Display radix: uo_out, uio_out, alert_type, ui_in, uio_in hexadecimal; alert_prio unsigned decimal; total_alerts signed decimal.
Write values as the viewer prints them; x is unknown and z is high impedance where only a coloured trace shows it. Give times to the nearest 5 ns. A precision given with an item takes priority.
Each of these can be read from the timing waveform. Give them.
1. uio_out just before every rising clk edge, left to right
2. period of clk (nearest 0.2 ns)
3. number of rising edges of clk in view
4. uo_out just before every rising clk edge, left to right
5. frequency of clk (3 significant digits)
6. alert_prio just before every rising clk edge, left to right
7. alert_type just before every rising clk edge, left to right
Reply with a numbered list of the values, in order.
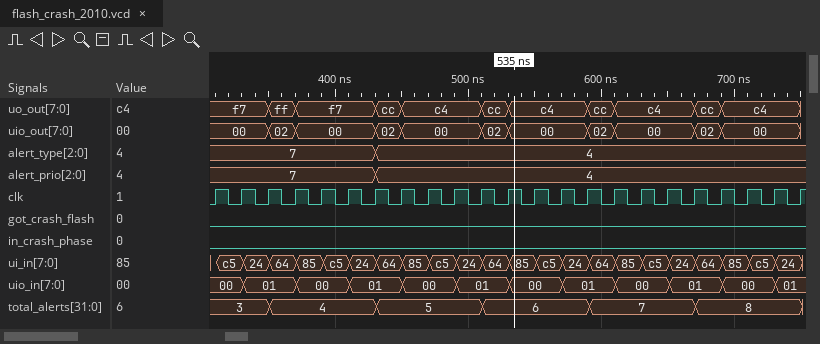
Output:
1. 00, 00, 00, 02, 00, 00, 00, 02, 00, 00, 00, 02, 00, 00, 00, 02, 00, 00, 00, 02, 00, 00, 00
2. 20 ns
3. 23
4. f7, f7, f7, ff, f7, f7, f7, cc, c4, c4, c4, cc, c4, c4, c4, cc, c4, c4, c4, cc, c4, c4, c4
5. 50.0 MHz
6. 7, 7, 7, 7, 7, 7, 7, 4, 4, 4, 4, 4, 4, 4, 4, 4, 4, 4, 4, 4, 4, 4, 4
7. 7, 7, 7, 7, 7, 7, 7, 4, 4, 4, 4, 4, 4, 4, 4, 4, 4, 4, 4, 4, 4, 4, 4
